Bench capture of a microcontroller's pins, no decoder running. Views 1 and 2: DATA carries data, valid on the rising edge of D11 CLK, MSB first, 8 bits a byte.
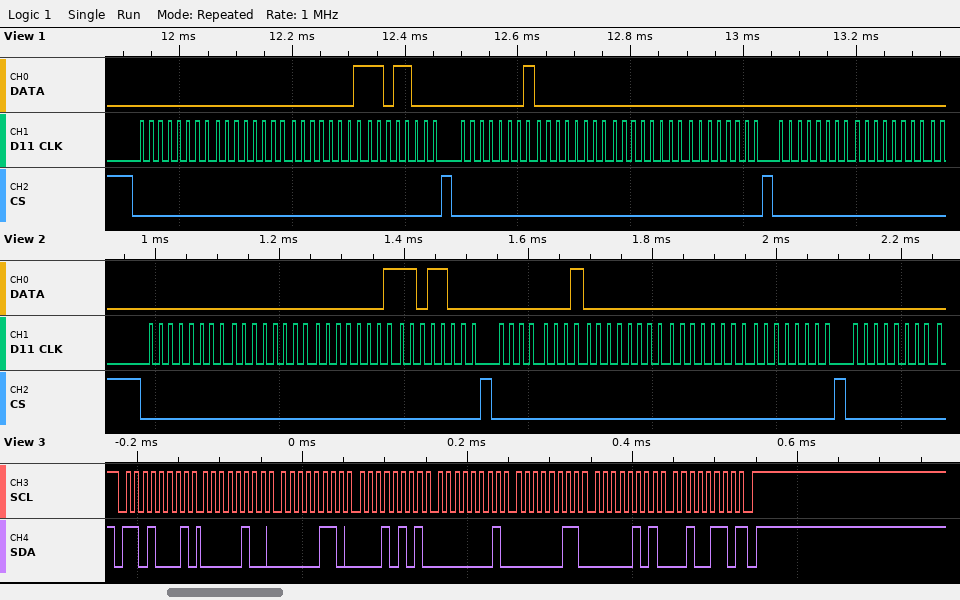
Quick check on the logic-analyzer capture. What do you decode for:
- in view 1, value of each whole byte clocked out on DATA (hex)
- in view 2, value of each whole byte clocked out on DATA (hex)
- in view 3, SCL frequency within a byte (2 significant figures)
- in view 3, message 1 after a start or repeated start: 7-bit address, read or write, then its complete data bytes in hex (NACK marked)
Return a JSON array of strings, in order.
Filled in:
["00 00 01 D8 01 00 00 00 00 00", "0x00 0x00 0x01 0xD8 0x01 0x00 0x00 0x00 0x00", "100 kHz", "0x68 read: 04 06 15 01 03 05 26 NACK"]
